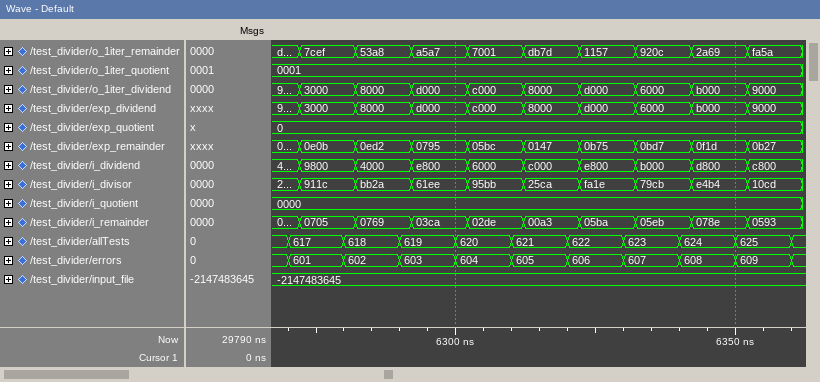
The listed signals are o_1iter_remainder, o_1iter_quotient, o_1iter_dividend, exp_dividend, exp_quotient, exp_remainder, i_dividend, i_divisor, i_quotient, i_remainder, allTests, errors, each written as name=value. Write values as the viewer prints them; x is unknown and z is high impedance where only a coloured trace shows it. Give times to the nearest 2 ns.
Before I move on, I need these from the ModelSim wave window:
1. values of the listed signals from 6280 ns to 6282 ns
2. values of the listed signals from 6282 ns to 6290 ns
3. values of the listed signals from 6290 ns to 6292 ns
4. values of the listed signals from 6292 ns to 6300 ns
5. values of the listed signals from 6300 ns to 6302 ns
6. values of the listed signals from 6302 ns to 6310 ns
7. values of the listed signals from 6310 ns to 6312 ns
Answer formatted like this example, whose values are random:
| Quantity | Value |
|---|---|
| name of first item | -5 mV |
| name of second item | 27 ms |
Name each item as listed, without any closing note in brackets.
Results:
| Quantity | Value |
|---|---|
| values of the listed signals from 6280 ns to 6282 ns | o_1iter_remainder=7cef, o_1iter_quotient=0001, o_1iter_dividend=3000, exp_dividend=3000, exp_quotient=0, exp_remainder=0e0b, i_dividend=9800, i_divisor=911c, i_quotient=0000, i_remainder=0705, allTests=618, errors=602 |
| values of the listed signals from 6282 ns to 6290 ns | o_1iter_remainder=53a8, o_1iter_quotient=0001, o_1iter_dividend=8000, exp_dividend=8000, exp_quotient=0, exp_remainder=0ed2, i_dividend=4000, i_divisor=bb2a, i_quotient=0000, i_remainder=0769, allTests=618, errors=602 |
| values of the listed signals from 6290 ns to 6292 ns | o_1iter_remainder=53a8, o_1iter_quotient=0001, o_1iter_dividend=8000, exp_dividend=8000, exp_quotient=0, exp_remainder=0ed2, i_dividend=4000, i_divisor=bb2a, i_quotient=0000, i_remainder=0769, allTests=619, errors=603 |
| values of the listed signals from 6292 ns to 6300 ns | o_1iter_remainder=a5a7, o_1iter_quotient=0001, o_1iter_dividend=d000, exp_dividend=d000, exp_quotient=0, exp_remainder=0795, i_dividend=e800, i_divisor=61ee, i_quotient=0000, i_remainder=03ca, allTests=619, errors=603 |
| values of the listed signals from 6300 ns to 6302 ns | o_1iter_remainder=a5a7, o_1iter_quotient=0001, o_1iter_dividend=d000, exp_dividend=d000, exp_quotient=0, exp_remainder=0795, i_dividend=e800, i_divisor=61ee, i_quotient=0000, i_remainder=03ca, allTests=620, errors=604 |
| values of the listed signals from 6302 ns to 6310 ns | o_1iter_remainder=7001, o_1iter_quotient=0001, o_1iter_dividend=c000, exp_dividend=c000, exp_quotient=0, exp_remainder=05bc, i_dividend=6000, i_divisor=95bb, i_quotient=0000, i_remainder=02de, allTests=620, errors=604 |
| values of the listed signals from 6310 ns to 6312 ns | o_1iter_remainder=7001, o_1iter_quotient=0001, o_1iter_dividend=c000, exp_dividend=c000, exp_quotient=0, exp_remainder=05bc, i_dividend=6000, i_divisor=95bb, i_quotient=0000, i_remainder=02de, allTests=621, errors=605 |
